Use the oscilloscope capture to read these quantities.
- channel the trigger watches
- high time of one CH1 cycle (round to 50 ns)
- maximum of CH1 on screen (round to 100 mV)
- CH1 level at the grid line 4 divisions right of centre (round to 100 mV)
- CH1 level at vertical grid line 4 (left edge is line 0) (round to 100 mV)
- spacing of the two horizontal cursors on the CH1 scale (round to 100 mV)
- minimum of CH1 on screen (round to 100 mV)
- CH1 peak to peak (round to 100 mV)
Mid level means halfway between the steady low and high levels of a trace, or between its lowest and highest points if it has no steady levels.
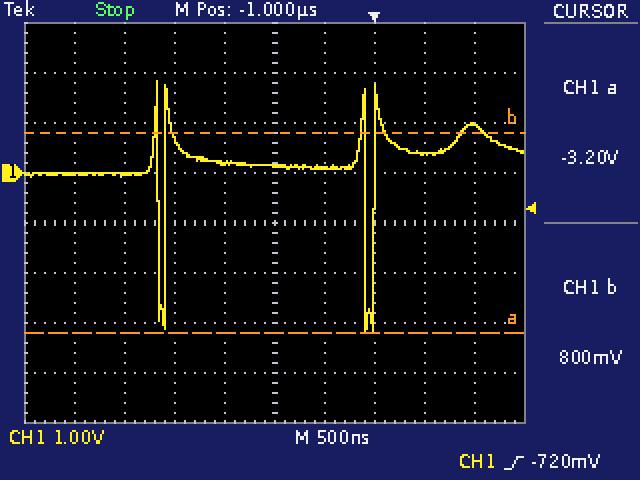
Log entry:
CH1
2.00 µs
1.8 V
1.0 V
200 mV
4.0 V
-3.2 V
5.0 V
